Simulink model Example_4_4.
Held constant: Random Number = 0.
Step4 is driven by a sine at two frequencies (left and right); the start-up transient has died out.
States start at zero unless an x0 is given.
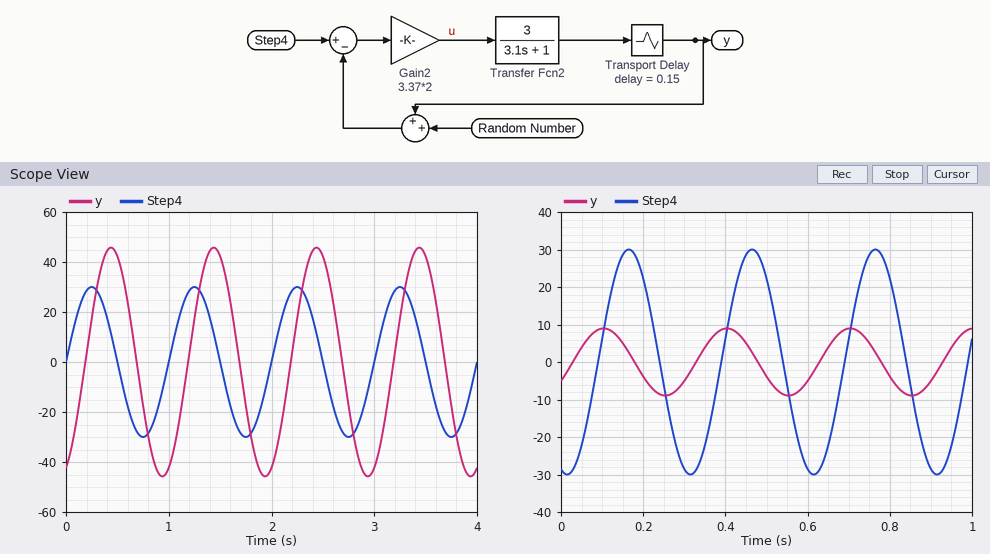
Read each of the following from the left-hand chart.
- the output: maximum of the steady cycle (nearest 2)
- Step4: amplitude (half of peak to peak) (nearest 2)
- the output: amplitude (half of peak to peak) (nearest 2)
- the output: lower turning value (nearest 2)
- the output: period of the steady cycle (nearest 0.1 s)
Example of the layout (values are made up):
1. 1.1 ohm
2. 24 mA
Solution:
1. 46
2. 30
3. 46
4. -46
5. 1.0 s
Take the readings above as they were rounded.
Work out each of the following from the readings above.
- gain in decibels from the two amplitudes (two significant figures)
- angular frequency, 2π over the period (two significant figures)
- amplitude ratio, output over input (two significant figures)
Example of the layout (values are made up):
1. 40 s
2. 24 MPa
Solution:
1. 3.7 dB
2. 6.3 rad/s
3. 1.5
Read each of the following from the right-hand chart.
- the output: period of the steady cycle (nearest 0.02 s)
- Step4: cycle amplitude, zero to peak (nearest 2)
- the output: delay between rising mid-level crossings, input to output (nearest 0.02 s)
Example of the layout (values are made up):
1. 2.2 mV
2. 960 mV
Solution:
1. 0.30 s
2. 30
3. 0.24 s
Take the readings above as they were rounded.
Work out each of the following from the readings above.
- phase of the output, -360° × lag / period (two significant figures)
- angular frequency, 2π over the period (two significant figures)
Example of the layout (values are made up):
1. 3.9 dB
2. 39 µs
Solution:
1. -290°
2. 21 rad/s
